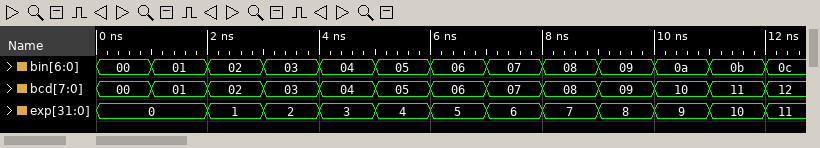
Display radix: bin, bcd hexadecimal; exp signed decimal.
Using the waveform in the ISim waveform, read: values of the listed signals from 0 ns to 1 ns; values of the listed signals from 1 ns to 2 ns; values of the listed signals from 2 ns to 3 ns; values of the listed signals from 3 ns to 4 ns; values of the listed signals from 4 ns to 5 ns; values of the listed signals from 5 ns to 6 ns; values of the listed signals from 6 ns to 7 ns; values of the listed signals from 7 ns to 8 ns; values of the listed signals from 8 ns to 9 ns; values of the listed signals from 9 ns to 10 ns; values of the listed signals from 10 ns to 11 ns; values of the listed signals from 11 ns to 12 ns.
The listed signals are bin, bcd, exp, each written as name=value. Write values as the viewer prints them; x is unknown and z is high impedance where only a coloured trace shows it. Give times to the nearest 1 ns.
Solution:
bin=00, bcd=00, exp=0
bin=01, bcd=01, exp=0
bin=02, bcd=02, exp=1
bin=03, bcd=03, exp=2
bin=04, bcd=04, exp=3
bin=05, bcd=05, exp=4
bin=06, bcd=06, exp=5
bin=07, bcd=07, exp=6
bin=08, bcd=08, exp=7
bin=09, bcd=09, exp=8
bin=0a, bcd=10, exp=9
bin=0b, bcd=11, exp=10
